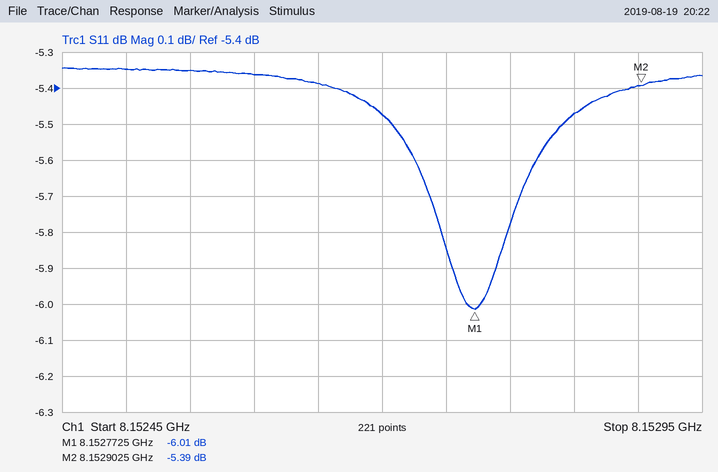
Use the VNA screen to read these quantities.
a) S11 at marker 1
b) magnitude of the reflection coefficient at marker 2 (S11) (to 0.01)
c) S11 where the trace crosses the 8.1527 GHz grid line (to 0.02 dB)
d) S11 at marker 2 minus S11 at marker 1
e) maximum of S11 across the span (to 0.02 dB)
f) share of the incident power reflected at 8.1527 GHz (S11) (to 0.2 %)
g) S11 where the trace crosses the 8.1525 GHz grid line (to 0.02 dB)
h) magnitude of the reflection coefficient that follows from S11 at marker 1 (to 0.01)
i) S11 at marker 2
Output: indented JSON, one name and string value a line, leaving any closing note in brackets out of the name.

{
  "S11 at marker 1": "-6.01 dB",
  "magnitude of the reflection coefficient at marker 2 (S11)": "0.54",
  "S11 where the trace crosses the 8.1527 GHz grid line": "-5.48 dB",
  "S11 at marker 2 minus S11 at marker 1": "0.62 dB",
  "maximum of S11 across the span": "-5.34 dB",
  "share of the incident power reflected at 8.1527 GHz (S11)": "28.4 %",
  "S11 where the trace crosses the 8.1525 GHz grid line": "-5.34 dB",
  "magnitude of the reflection coefficient that follows from S11 at marker 1": "0.50",
  "S11 at marker 2": "-5.39 dB"
}
